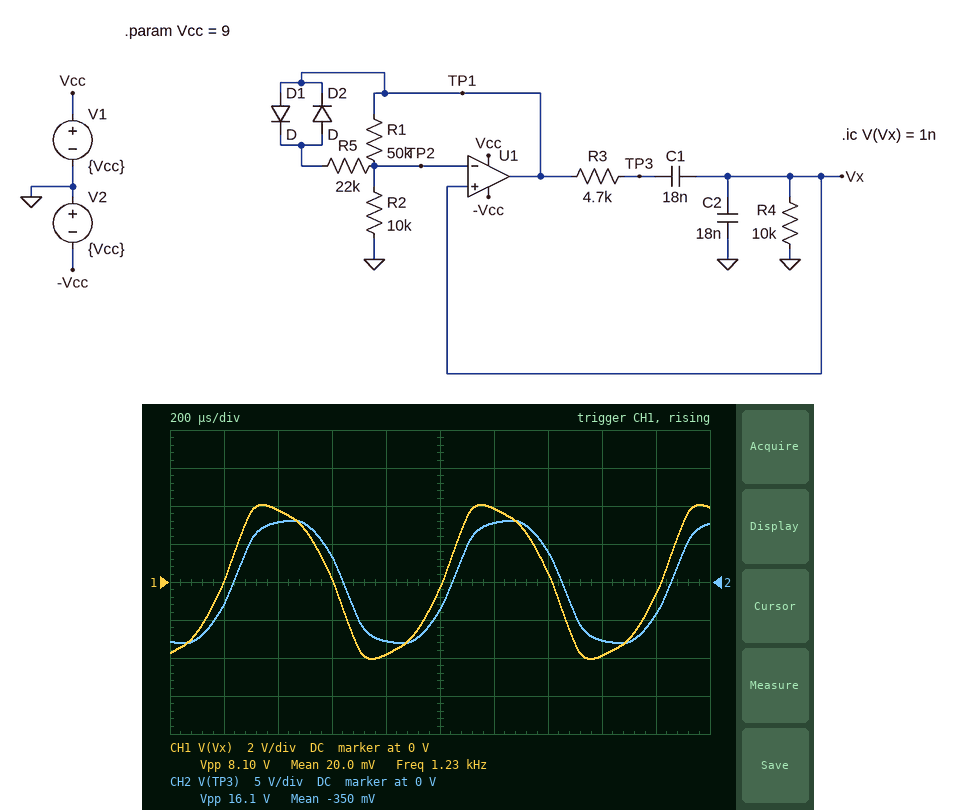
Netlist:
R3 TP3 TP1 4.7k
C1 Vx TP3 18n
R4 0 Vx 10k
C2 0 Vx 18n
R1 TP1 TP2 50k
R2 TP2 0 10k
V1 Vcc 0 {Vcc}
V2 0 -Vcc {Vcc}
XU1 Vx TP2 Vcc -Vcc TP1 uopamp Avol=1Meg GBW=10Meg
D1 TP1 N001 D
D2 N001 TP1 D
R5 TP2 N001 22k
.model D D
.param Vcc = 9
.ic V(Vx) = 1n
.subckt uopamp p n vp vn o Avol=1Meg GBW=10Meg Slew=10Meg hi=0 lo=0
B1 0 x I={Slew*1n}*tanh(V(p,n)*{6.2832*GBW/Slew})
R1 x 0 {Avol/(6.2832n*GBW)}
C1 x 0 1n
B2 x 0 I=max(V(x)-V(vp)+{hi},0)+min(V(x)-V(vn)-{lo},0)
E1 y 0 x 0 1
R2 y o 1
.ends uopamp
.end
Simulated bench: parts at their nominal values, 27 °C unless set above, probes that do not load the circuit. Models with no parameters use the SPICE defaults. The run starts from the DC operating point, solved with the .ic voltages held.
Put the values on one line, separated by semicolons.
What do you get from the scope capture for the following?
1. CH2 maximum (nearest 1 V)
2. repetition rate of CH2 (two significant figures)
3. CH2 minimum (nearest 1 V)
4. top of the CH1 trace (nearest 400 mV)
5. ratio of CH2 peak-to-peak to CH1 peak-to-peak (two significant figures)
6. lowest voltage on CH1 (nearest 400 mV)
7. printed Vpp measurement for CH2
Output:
8 V; 1.2 kHz; -8 V; 4.0 V; 2.0; -4.0 V; 16.1 V
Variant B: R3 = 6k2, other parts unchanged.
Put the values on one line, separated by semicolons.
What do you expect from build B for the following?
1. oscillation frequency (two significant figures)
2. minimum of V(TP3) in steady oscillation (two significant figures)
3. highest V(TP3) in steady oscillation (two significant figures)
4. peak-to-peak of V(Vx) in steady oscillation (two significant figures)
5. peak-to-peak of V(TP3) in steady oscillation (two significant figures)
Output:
1.1 kHz; -7.6 V; 7.6 V; 7.3 V; 15 V
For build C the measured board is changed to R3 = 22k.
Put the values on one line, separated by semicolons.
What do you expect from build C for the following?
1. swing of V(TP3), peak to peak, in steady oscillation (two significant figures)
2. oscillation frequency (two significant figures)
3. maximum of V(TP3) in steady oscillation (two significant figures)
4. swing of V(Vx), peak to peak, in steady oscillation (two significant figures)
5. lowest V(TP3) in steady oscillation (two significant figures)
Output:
1.3 V; 570 Hz; 640 mV; 550 mV; -640 mV
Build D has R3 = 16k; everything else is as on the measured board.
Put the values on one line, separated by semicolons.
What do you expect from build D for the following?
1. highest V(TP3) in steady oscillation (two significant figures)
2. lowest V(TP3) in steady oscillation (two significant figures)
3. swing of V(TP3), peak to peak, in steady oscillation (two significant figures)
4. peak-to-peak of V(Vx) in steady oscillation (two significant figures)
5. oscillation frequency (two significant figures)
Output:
1.0 V; -1.0 V; 2.0 V; 900 mV; 670 Hz
